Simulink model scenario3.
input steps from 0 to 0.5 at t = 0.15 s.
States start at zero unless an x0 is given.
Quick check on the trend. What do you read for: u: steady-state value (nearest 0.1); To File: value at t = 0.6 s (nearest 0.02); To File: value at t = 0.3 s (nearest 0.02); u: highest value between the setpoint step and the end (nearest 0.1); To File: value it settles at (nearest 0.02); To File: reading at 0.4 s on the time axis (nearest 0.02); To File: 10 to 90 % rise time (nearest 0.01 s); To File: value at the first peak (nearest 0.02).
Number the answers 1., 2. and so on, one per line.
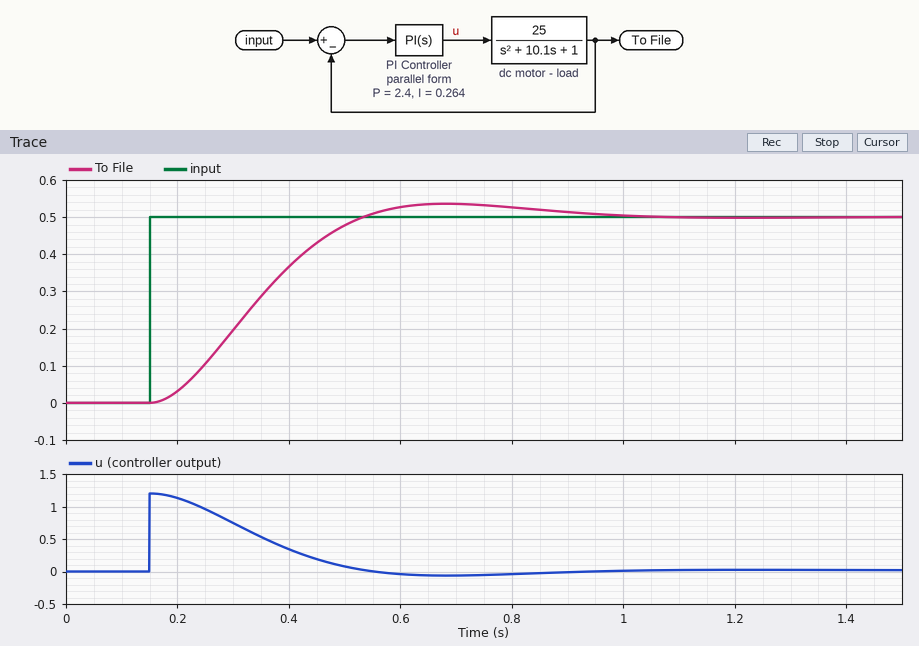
1. 0.0
2. 0.52
3. 0.20
4. 1.2
5. 0.50
6. 0.36
7. 0.25 s
8. 0.54
